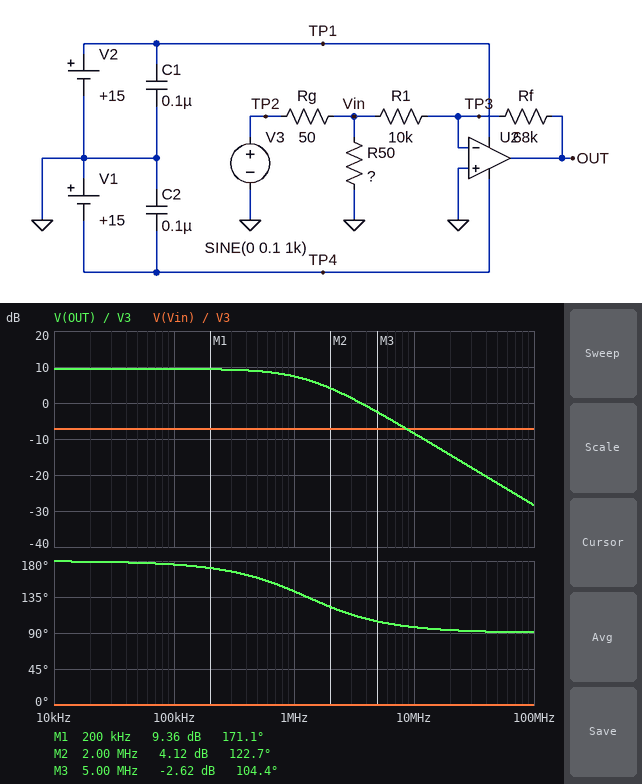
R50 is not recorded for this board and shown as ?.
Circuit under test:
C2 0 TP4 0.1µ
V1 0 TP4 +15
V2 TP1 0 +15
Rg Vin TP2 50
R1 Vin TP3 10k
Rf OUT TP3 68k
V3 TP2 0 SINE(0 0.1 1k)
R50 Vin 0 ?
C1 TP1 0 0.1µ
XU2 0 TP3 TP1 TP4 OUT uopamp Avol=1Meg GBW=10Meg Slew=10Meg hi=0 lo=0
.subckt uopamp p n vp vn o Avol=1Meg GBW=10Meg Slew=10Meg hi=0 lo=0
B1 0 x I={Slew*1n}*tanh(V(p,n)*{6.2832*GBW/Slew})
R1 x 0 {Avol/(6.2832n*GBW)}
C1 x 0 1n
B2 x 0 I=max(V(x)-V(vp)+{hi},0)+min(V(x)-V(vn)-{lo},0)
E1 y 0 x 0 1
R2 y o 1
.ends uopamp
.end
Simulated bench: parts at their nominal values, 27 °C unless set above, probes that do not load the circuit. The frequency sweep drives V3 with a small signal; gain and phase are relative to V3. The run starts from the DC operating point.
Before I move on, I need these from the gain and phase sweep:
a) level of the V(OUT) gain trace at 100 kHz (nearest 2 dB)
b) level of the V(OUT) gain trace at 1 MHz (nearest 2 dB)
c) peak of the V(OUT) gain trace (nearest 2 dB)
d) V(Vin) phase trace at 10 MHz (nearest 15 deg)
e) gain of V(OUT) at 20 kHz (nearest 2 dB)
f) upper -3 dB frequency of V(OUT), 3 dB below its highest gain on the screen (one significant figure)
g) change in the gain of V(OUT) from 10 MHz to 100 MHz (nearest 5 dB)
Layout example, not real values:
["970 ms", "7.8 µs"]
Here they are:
["10 dB", "8 dB", "10 dB", "0 deg", "10 dB", "1 MHz", "-20 dB"]
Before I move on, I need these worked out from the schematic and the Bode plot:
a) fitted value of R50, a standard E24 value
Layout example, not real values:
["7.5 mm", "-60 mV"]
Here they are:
["39 Ω"]
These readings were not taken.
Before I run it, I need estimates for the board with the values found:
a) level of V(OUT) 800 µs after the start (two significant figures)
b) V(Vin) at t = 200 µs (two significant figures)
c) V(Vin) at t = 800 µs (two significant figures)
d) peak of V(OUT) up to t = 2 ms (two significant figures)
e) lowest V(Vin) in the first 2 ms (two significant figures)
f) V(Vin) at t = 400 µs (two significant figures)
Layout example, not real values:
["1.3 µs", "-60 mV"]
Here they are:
["280 mV", "42 mV", "-42 mV", "300 mV", "-44 mV", "26 mV"]
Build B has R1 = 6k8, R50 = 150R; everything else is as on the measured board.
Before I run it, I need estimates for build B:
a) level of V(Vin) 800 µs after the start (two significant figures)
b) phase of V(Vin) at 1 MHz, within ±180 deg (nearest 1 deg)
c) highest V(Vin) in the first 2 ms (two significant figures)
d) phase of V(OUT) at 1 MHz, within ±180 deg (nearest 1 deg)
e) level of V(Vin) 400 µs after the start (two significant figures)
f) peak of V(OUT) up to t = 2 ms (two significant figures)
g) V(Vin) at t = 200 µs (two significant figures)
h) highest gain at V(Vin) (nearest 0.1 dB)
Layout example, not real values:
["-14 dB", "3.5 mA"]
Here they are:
["-71 mV", "0 deg", "75 mV", "132 deg", "44 mV", "750 mV", "71 mV", "-2.5 dB"]
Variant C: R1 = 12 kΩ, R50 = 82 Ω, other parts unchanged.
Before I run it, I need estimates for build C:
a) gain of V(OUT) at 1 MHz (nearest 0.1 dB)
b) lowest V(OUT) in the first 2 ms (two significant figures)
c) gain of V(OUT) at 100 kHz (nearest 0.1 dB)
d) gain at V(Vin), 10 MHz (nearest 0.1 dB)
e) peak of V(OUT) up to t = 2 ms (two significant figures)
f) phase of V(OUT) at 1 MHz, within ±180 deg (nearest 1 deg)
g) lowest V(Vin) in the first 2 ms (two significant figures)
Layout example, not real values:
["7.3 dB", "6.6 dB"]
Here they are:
["9.3 dB", "-350 mV", "10.9 dB", "-4.1 dB", "350 mV", "146 deg", "-62 mV"]
